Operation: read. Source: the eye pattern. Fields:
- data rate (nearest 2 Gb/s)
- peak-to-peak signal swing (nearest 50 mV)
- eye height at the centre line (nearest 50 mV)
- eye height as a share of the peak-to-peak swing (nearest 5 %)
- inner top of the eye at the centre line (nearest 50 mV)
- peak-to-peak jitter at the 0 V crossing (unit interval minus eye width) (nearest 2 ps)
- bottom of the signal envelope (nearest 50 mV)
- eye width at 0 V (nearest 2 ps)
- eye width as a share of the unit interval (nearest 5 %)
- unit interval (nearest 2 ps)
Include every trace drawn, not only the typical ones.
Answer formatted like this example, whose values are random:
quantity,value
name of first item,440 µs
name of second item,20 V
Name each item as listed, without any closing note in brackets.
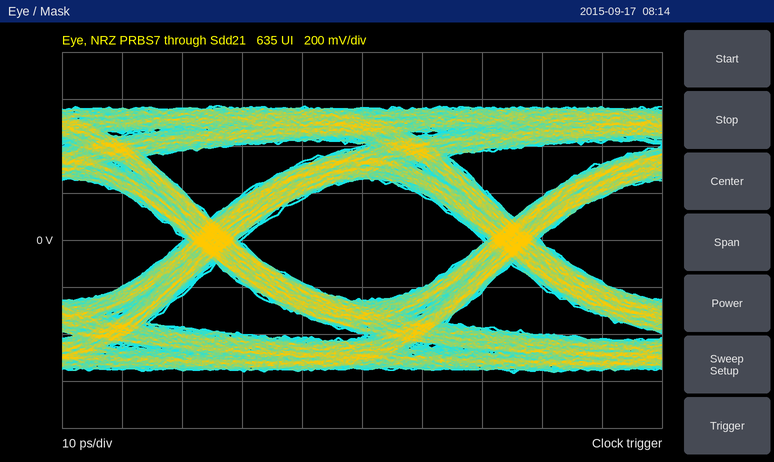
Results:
quantity,value
data rate,20 Gb/s
peak-to-peak signal swing,1.15 V
eye height at the centre line,500 mV
eye height as a share of the peak-to-peak swing,45 %
inner top of the eye at the centre line,250 mV
peak-to-peak jitter at the 0 V crossing (unit interval minus eye width),10 ps
bottom of the signal envelope,-550 mV
eye width at 0 V,40 ps
eye width as a share of the unit interval,80 %
unit interval,50 ps
